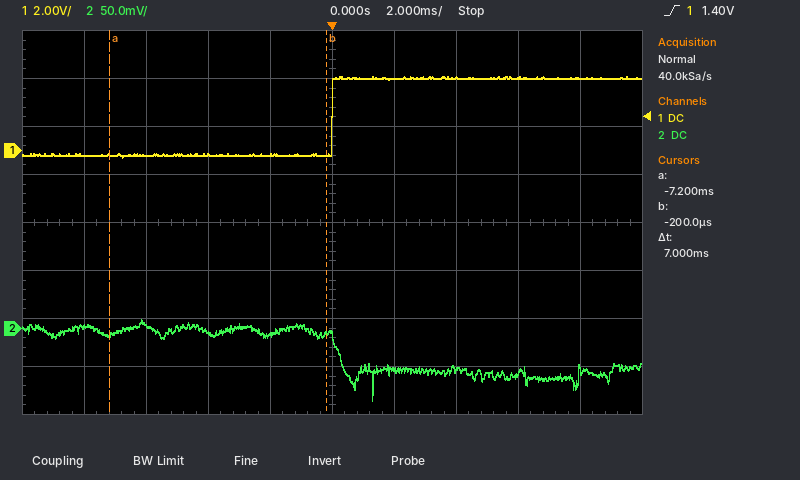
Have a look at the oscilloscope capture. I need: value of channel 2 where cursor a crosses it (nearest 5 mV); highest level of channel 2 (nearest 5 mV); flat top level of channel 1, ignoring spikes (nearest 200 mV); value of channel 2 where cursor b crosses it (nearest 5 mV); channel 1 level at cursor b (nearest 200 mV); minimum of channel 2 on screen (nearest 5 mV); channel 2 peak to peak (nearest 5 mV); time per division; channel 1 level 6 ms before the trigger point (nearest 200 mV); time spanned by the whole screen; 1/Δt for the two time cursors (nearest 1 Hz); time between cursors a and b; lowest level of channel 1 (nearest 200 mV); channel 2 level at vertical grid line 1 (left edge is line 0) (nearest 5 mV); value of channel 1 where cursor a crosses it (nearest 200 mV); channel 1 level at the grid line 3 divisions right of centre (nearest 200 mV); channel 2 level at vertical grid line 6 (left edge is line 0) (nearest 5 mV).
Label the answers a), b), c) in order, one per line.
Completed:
a) -5 mV
b) 10 mV
c) 3.0 V
d) -5 mV
e) -200 mV
f) -75 mV
g) 85 mV
h) 2 ms
i) -200 mV
j) 20 ms
k) 143 Hz
l) 7 ms
m) -200 mV
n) 0 mV
o) -200 mV
p) 3.0 V
q) -45 mV
